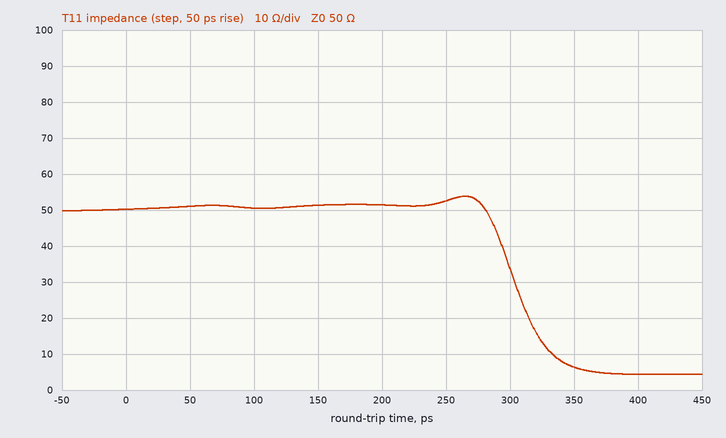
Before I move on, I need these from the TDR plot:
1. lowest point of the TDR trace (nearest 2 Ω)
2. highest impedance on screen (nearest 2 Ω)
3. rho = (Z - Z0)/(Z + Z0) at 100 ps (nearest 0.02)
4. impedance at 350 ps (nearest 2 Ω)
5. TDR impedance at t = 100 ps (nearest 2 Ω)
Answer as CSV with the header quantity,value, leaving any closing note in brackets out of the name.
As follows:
quantity,value
lowest point of the TDR trace,4 Ω
highest impedance on screen,54 Ω
rho = (Z - Z0)/(Z + Z0) at 100 ps,0.00
impedance at 350 ps,6 Ω
TDR impedance at t = 100 ps,50 Ω
